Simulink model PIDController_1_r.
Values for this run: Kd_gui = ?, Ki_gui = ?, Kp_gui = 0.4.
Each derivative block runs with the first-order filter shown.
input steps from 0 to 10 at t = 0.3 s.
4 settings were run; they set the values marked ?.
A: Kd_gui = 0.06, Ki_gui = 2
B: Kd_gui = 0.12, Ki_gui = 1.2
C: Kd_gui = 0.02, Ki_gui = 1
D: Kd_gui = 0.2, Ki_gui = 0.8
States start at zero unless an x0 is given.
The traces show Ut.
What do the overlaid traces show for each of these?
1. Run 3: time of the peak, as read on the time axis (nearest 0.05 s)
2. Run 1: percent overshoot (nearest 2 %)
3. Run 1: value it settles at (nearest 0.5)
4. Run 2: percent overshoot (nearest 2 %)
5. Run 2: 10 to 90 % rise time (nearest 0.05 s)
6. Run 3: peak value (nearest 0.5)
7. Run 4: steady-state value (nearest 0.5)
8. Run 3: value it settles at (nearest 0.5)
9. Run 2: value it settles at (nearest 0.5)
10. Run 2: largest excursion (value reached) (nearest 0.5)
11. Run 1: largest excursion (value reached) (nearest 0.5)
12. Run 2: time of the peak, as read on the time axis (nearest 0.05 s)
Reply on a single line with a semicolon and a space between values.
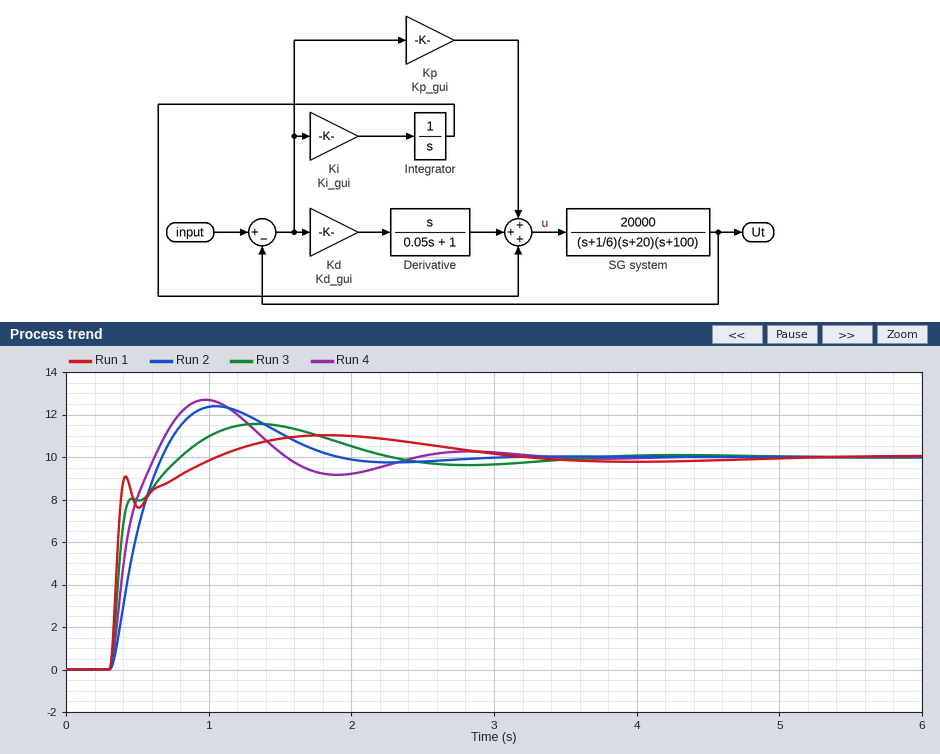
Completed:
1.35 s; 10 %; 10.0; 24 %; 0.25 s; 11.5; 10.0; 10.0; 10.0; 12.5; 11.0; 1.05 s
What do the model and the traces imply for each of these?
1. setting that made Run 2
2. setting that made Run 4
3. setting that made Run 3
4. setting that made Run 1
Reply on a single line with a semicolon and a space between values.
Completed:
C; A; B; D
